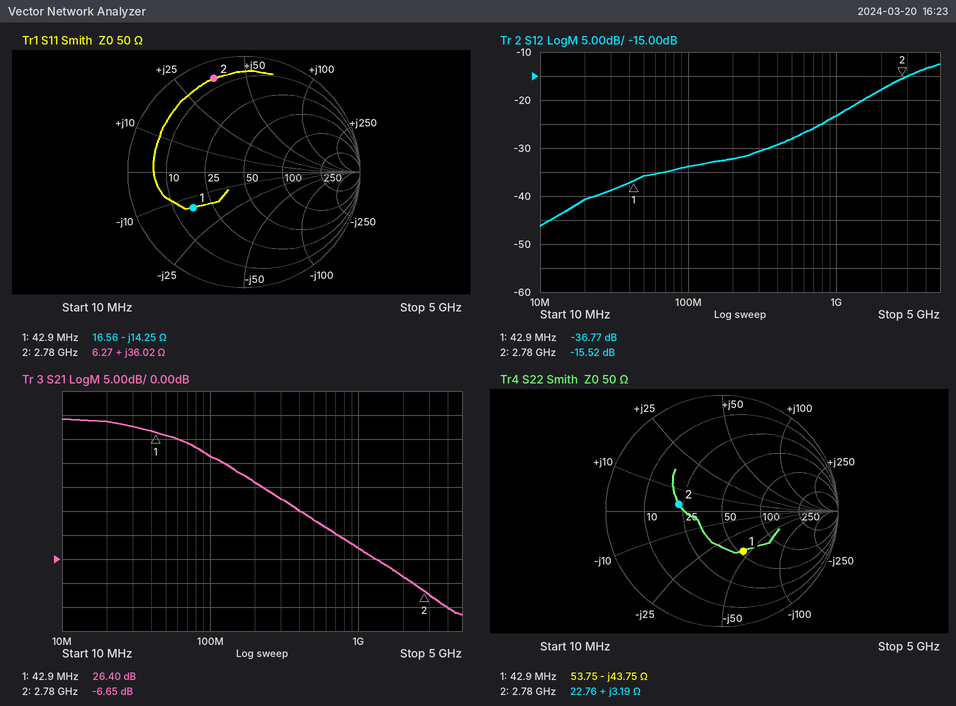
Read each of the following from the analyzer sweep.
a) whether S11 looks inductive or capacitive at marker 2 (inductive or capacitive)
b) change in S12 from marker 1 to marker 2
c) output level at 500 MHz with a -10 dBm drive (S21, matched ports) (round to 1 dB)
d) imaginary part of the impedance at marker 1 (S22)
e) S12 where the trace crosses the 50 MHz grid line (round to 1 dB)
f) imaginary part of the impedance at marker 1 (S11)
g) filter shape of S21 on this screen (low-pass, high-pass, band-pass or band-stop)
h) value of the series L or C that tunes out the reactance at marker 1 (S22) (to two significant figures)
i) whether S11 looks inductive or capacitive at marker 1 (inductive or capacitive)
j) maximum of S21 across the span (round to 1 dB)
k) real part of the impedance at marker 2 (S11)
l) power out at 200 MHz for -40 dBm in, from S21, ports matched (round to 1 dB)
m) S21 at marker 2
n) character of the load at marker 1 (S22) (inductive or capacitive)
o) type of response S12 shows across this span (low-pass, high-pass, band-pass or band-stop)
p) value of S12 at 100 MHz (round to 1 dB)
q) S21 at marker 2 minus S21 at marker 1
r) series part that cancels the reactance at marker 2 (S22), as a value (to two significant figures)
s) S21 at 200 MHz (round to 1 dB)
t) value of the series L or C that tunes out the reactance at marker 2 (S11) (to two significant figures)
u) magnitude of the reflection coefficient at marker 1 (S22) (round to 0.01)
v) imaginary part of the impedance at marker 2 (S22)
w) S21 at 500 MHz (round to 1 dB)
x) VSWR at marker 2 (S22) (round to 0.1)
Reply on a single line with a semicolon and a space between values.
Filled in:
inductive; 21.25 dB; -2 dBm; -43.75 Ω; -36 dB; -14.25 Ω; low-pass; 160 nH; capacitive; 29 dB; 6.27 Ω; -24 dBm; -6.65 dB; capacitive; high-pass; -34 dB; -33.05 dB; 18 pF; 16 dB; 1.6 pF; 0.39; +3.19 Ω; 8 dB; 2.2
